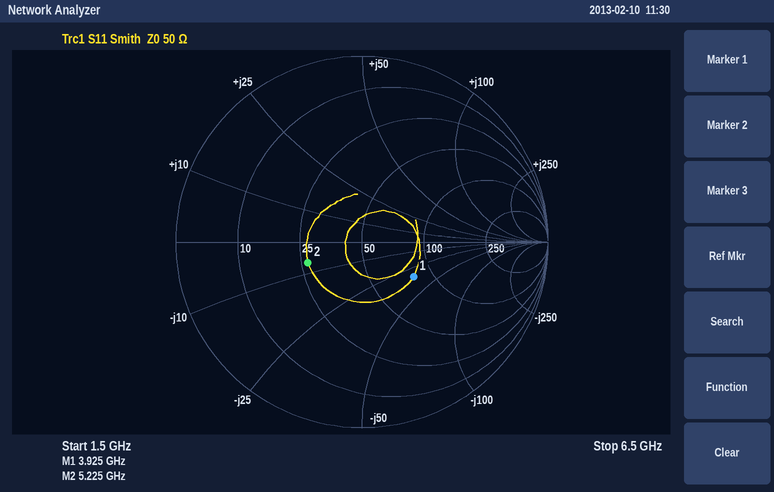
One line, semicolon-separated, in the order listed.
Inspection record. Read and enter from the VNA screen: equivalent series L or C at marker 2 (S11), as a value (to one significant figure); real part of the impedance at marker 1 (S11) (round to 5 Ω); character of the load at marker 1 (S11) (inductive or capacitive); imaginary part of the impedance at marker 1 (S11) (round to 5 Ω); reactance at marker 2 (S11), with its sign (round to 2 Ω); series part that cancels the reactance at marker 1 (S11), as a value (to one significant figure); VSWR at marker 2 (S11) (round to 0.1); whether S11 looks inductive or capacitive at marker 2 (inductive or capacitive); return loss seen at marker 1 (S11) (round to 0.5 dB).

5 pF; 80 Ω; capacitive; -35 Ω; -6 Ω; 1 nH; 1.9; capacitive; 9.5 dB
